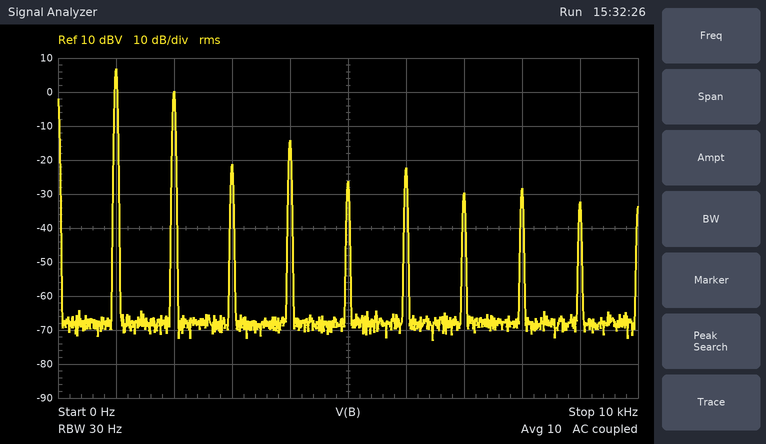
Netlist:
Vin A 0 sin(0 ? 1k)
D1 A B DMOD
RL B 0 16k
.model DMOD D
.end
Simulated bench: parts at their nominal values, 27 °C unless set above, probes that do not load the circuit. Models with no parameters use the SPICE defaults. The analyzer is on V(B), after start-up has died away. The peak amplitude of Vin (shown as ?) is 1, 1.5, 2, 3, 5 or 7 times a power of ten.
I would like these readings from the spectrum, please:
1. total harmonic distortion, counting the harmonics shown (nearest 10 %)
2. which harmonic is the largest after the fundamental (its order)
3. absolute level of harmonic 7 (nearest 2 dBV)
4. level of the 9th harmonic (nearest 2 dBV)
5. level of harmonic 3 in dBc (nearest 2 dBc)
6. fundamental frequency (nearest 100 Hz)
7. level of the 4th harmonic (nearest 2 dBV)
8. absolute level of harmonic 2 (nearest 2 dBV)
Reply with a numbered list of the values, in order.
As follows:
1. 50 %
2. 2
3. -30 dBV
4. -32 dBV
5. -28 dBc
6. 1.0 kHz
7. -14 dBV
8. 0 dBV
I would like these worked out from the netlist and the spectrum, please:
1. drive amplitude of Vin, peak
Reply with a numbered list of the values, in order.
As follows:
1. 7 V
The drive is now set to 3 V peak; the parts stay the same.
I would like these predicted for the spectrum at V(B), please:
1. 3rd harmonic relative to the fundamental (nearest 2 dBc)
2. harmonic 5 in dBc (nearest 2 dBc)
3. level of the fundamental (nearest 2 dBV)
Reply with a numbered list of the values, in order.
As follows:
1. -20 dBc
2. -26 dBc
3. -2 dBV
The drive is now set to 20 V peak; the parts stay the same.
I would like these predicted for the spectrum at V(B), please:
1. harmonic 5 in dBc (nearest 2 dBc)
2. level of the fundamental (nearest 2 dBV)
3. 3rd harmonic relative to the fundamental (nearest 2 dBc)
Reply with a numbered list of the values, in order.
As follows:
1. -42 dBc
2. 16 dBV
3. -38 dBc
